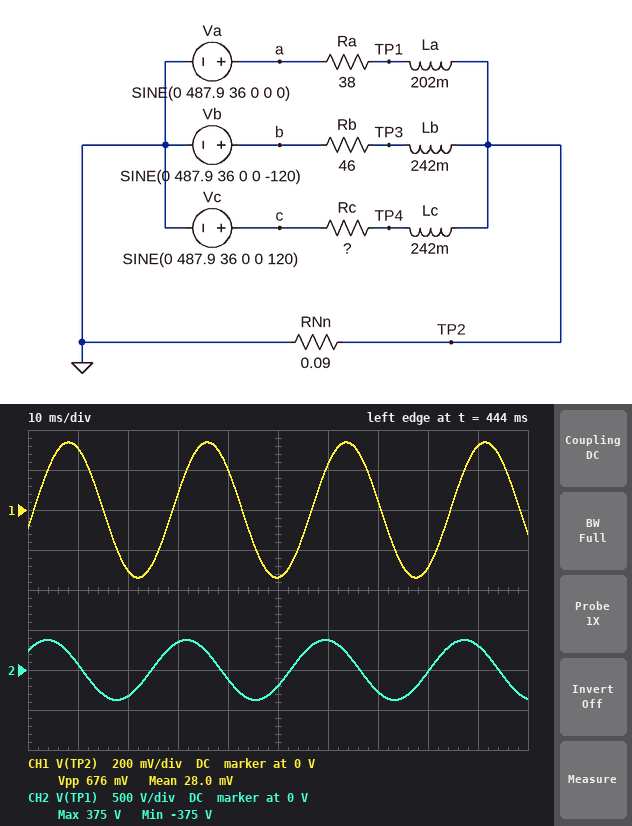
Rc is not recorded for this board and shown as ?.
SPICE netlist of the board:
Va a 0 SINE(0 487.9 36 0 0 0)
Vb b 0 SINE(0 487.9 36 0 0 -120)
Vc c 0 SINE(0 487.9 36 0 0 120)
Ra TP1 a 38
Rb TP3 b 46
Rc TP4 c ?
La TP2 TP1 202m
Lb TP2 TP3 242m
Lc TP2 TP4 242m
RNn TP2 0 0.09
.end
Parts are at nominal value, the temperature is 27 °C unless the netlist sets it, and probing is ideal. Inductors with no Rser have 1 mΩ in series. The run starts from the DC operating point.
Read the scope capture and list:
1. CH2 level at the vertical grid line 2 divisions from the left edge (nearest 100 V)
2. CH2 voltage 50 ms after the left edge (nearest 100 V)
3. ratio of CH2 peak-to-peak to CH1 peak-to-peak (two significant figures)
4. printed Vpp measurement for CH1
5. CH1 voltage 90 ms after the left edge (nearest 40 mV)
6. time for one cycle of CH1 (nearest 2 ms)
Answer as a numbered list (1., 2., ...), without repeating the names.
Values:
1. -300 V
2. -200 V
3. 1100
4. 676 mV
5. 320 mV
6. 28 ms
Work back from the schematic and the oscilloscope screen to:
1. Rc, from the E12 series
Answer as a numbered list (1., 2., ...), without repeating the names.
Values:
1. 22 Ω
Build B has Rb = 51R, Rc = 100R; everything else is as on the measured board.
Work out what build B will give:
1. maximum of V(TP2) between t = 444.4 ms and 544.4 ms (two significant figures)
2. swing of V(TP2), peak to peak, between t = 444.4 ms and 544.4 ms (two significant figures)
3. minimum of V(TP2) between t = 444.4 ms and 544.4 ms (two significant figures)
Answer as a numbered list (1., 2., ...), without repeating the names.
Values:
1. 330 mV
2. 660 mV
3. -330 mV
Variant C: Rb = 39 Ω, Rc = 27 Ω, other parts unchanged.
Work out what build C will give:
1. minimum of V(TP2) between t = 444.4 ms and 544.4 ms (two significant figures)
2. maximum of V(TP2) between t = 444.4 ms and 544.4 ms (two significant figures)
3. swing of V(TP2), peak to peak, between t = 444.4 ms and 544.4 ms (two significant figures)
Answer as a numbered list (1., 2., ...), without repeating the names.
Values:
1. -220 mV
2. 220 mV
3. 450 mV
